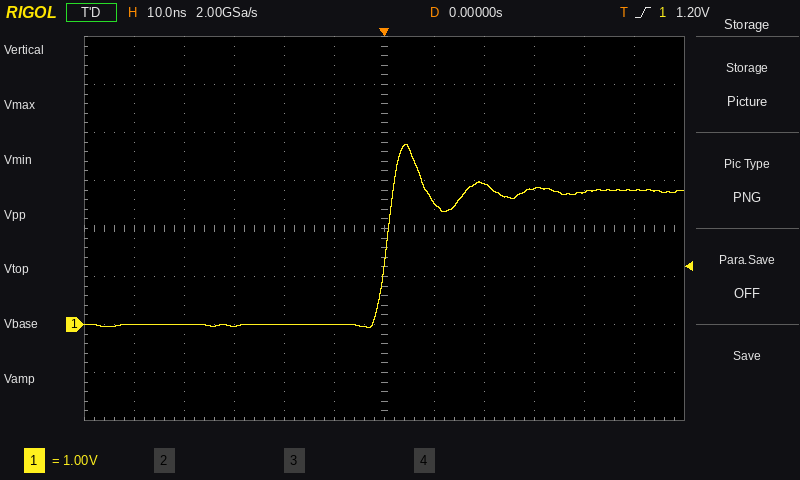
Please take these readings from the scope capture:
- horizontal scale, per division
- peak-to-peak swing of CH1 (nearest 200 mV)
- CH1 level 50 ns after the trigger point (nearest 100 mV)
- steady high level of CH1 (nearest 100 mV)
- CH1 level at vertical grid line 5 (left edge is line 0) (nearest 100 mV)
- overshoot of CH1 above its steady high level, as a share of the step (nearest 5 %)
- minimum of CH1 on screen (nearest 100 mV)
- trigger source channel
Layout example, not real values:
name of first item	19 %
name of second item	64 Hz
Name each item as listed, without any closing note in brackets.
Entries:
horizontal scale, per division	10 ns
peak-to-peak swing of CH1	3.8 V
CH1 level 50 ns after the trigger point	2.8 V
steady high level of CH1	2.8 V
CH1 level at vertical grid line 5 (left edge is line 0)	0.0 V
overshoot of CH1 above its steady high level, as a share of the step	35 %
minimum of CH1 on screen	-100 mV
trigger source channel	CH1
